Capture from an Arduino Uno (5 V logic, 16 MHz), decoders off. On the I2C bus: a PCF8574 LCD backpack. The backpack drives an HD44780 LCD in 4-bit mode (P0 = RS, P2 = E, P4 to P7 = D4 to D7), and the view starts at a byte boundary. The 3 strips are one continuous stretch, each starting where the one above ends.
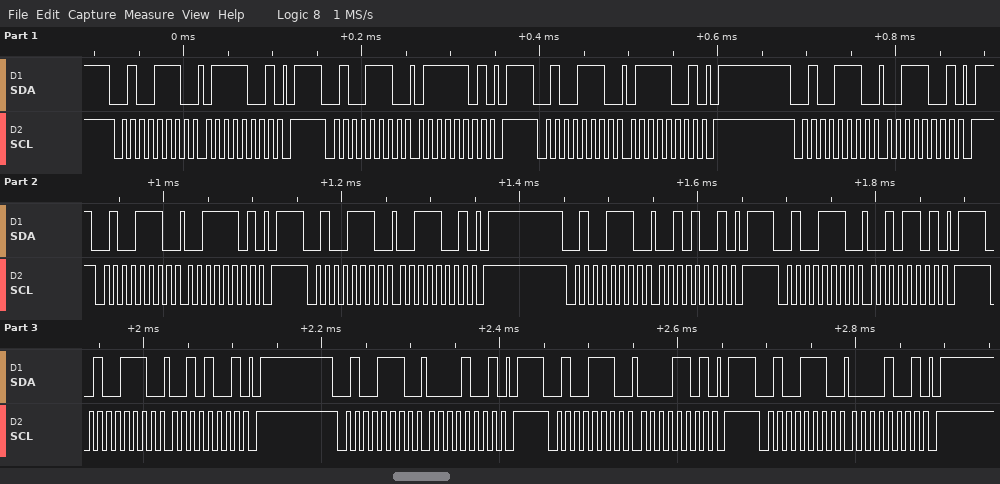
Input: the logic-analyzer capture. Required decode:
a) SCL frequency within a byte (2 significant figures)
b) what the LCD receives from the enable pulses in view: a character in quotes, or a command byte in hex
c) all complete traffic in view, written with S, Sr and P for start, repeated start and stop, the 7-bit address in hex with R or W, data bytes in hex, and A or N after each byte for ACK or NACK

100 kHz
's' ' '
S 27W A 79 A P S 27W A 7D A P S 27W A 79 A P S 27W A 39 A P S 27W A 3D A P S 27W A 39 A P S 27W A 29 A P S 27W A 2D A P S 27W A 29 A P S 27W A 09 A P S 27W A 0D A P S 27W A 09 A P
